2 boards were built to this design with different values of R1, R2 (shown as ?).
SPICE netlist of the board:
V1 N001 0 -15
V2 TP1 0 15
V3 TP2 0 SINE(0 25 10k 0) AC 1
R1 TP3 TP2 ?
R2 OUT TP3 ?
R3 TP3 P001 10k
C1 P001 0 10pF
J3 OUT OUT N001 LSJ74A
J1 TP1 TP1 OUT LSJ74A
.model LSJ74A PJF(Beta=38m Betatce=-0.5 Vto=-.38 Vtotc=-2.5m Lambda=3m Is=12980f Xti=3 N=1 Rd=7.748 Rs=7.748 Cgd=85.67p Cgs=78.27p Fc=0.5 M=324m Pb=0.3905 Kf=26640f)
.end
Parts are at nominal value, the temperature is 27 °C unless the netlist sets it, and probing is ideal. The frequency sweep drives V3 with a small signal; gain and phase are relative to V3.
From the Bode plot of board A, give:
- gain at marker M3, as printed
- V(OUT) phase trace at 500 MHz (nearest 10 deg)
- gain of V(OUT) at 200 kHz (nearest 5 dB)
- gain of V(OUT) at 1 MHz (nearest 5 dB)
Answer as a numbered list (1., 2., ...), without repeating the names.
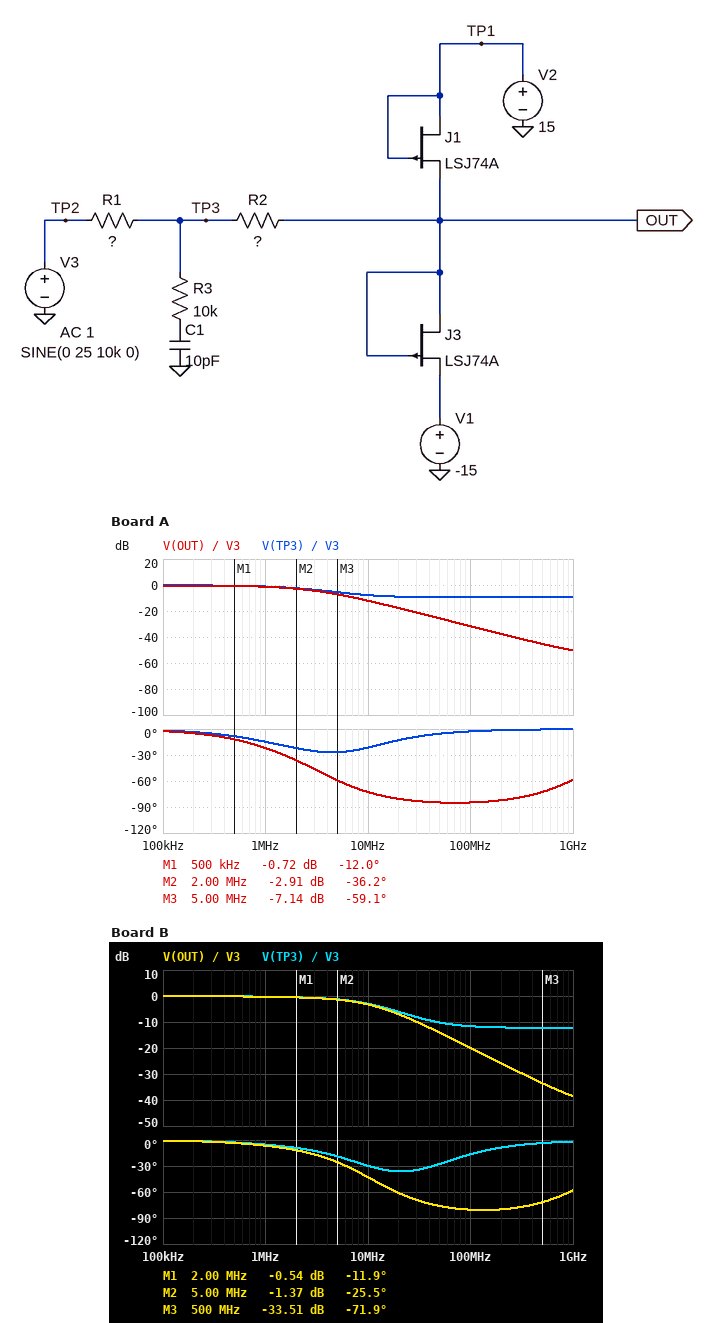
1. -7.14 dB
2. -70 deg
3. 0 dB
4. 0 dB
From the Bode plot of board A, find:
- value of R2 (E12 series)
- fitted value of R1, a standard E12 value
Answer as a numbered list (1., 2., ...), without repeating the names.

1. 820 Ω
2. 1.5 kΩ
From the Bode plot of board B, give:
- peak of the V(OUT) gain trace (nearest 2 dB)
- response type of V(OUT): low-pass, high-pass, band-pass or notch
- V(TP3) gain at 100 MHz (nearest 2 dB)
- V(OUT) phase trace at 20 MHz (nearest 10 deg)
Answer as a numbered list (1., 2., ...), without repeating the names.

1. 0 dB
2. low-pass
3. -12 dB
4. -60 deg
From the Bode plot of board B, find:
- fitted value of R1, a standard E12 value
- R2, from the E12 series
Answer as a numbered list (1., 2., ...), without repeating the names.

1. 470 Ω
2. 150 Ω
